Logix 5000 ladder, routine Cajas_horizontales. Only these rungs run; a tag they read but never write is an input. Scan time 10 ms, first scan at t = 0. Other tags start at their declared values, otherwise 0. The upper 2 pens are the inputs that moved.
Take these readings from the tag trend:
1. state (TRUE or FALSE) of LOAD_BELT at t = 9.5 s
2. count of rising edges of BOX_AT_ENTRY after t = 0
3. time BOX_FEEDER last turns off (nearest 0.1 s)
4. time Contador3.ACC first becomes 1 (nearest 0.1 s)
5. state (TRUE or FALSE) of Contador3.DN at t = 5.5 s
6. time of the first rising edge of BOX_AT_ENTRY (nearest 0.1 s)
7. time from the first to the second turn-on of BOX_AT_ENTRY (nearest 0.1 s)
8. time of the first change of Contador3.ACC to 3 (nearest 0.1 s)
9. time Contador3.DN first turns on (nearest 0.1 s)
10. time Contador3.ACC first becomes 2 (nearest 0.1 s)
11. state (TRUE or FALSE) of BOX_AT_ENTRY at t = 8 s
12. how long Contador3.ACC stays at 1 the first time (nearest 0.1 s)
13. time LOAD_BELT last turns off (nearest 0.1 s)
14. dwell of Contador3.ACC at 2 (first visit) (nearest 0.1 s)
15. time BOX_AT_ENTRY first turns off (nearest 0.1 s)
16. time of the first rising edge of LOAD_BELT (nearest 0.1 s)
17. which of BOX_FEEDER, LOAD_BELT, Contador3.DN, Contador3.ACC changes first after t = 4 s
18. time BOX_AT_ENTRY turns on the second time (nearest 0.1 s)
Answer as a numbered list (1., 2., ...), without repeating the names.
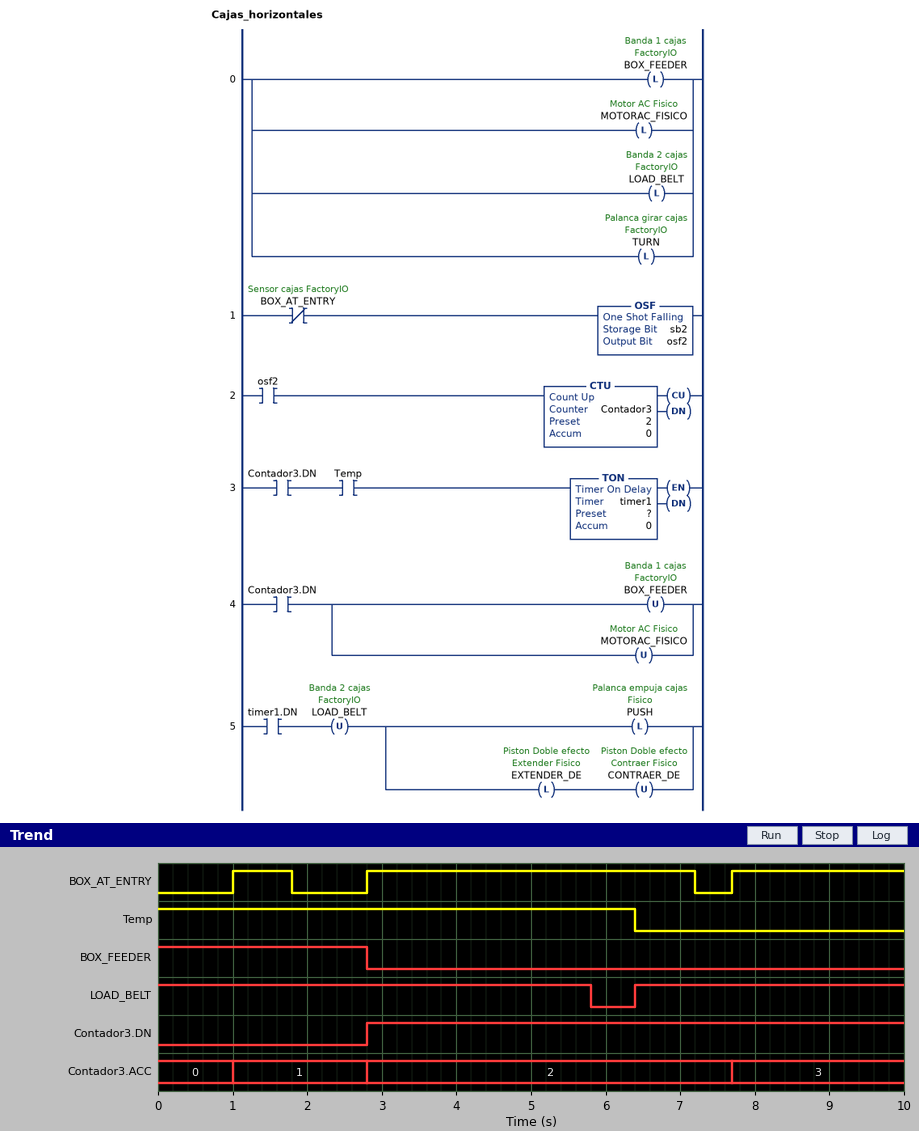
1. TRUE
2. 3
3. 2.8 s
4. 1.0 s
5. TRUE
6. 1.0 s
7. 1.8 s
8. 7.7 s
9. 2.8 s
10. 2.8 s
11. TRUE
12. 1.8 s
13. 5.8 s
14. 4.9 s
15. 1.8 s
16. 6.4 s
17. LOAD_BELT
18. 2.8 s
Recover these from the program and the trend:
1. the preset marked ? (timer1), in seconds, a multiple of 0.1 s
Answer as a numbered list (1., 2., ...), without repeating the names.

1. 3.0 s
